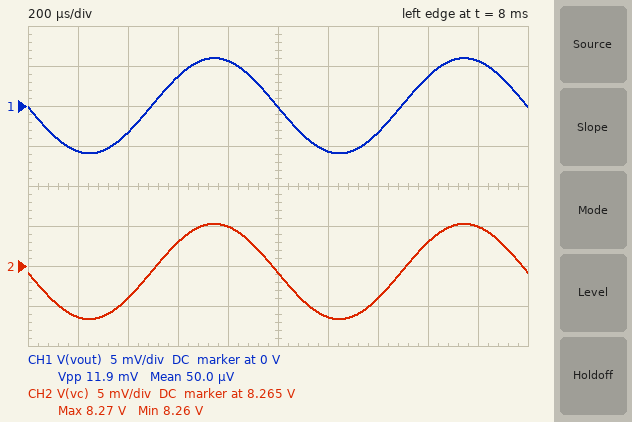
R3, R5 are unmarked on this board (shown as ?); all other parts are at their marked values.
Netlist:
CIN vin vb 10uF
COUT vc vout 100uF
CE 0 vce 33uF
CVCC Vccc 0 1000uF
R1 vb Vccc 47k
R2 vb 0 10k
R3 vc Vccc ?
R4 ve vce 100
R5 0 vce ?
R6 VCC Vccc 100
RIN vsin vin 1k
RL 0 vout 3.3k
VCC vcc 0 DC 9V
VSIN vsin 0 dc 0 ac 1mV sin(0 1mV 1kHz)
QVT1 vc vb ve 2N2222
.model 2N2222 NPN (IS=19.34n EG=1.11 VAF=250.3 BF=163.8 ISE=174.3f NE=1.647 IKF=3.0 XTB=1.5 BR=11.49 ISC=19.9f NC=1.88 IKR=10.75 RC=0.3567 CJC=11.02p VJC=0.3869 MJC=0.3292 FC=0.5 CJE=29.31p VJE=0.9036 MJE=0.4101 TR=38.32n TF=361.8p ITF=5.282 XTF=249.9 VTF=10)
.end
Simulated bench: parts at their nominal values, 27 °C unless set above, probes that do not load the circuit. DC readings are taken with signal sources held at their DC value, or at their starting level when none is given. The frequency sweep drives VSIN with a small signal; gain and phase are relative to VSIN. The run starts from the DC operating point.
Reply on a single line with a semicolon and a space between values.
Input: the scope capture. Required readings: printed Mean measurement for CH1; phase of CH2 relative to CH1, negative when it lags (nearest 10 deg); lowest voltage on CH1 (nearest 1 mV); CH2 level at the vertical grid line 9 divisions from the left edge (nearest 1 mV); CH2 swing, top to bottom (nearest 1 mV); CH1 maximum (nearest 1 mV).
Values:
50.0 µV; 0 deg; -6 mV; 8.270 V; 12 mV; 6 mV
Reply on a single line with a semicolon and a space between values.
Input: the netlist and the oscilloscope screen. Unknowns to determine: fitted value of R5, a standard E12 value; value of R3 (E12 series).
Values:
3.3 kΩ; 1.8 kΩ
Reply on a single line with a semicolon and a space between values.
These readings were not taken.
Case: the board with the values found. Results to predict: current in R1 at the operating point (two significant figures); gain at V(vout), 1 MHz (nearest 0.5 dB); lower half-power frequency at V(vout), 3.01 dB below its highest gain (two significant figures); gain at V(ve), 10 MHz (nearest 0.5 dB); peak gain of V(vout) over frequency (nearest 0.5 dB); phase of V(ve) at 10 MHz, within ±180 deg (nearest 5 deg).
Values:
160 µA; 15.0 dB; 30 Hz; -15.0 dB; 15.5 dB; -50 deg
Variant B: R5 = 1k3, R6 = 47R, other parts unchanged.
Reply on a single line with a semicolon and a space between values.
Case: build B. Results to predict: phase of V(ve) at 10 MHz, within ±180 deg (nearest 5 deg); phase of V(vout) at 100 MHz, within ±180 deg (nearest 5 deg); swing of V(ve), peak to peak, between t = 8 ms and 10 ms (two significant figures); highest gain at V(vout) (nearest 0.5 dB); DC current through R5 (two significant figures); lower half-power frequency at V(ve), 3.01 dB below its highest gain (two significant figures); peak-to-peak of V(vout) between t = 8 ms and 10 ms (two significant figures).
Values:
-55 deg; 40 deg; 1.3 mV; 17.5 dB; 890 µA; 1.7 Hz; 15 mV
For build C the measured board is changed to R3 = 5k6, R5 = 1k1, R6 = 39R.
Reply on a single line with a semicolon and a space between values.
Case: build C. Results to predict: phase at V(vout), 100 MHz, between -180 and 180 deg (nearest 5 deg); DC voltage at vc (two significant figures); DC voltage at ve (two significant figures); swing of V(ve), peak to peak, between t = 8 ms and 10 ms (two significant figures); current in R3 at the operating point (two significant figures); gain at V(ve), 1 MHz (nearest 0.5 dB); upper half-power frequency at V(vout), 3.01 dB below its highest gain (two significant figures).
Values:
35 deg; 3.2 V; 1.2 V; 1.4 mV; 1.0 mA; -5.0 dB; 1.4 MHz
